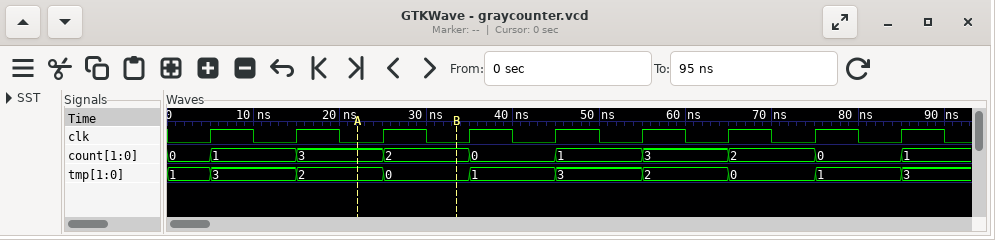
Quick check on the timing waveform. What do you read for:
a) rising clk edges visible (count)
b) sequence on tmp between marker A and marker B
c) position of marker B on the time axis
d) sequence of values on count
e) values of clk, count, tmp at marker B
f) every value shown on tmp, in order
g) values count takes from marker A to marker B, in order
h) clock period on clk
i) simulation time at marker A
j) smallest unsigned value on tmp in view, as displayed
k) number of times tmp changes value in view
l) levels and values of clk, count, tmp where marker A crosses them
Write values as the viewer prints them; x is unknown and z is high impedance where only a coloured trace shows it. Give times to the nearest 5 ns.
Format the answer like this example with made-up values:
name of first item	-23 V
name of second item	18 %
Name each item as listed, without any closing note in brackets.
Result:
rising clk edges visible	9
sequence on tmp between marker A and marker B	2, 0
position of marker B on the time axis	35 ns
sequence of values on count	0, 1, 3, 2, 0, 1, 3, 2, 0, 1
values of clk, count, tmp at marker B	clk=0, count=2, tmp=0
every value shown on tmp, in order	1, 3, 2, 0, 1, 3, 2, 0, 1, 3
values count takes from marker A to marker B, in order	3, 2
clock period on clk	10 ns
simulation time at marker A	20 ns
smallest unsigned value on tmp in view, as displayed	0
number of times tmp changes value in view	9
levels and values of clk, count, tmp where marker A crosses them	clk=0, count=3, tmp=2
